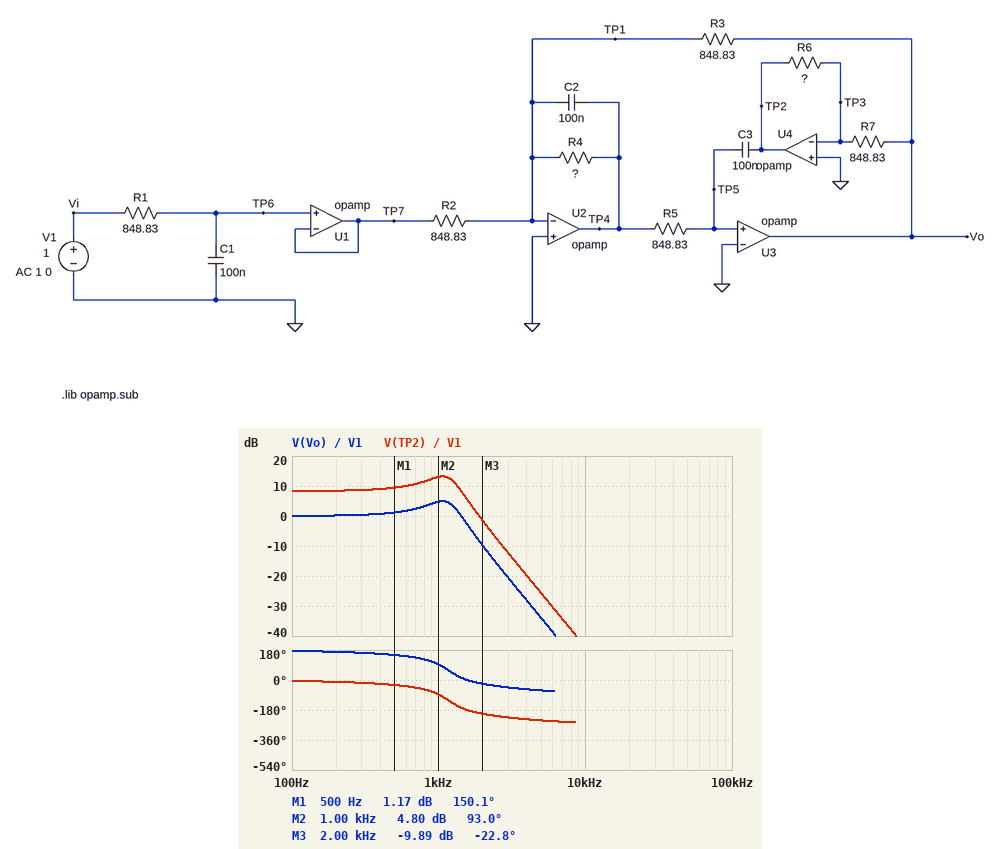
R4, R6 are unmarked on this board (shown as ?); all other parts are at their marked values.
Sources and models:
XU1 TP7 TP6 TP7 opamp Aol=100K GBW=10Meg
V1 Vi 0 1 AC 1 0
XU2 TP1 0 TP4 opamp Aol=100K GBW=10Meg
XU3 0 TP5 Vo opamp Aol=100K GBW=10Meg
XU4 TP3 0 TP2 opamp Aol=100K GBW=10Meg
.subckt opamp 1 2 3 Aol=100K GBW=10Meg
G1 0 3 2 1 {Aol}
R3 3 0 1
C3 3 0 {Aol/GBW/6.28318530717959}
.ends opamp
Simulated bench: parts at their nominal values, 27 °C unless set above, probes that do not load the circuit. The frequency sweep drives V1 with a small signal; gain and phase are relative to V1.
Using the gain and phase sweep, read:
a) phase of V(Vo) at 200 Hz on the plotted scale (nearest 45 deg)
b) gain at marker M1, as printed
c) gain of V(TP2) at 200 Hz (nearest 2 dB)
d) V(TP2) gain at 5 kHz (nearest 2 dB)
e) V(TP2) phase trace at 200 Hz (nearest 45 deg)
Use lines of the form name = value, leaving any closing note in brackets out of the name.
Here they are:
phase of V(Vo) at 200 Hz on the plotted scale = 180 deg
gain at marker M1, as printed = 1.17 dB
gain of V(TP2) at 200 Hz = 8 dB
V(TP2) gain at 5 kHz = -26 dB
V(TP2) phase trace at 200 Hz = 0 deg
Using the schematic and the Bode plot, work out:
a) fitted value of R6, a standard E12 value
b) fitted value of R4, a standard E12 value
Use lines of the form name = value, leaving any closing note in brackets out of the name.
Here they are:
fitted value of R6, a standard E12 value = 2.2 kΩ
fitted value of R4, a standard E12 value = 2.7 kΩ
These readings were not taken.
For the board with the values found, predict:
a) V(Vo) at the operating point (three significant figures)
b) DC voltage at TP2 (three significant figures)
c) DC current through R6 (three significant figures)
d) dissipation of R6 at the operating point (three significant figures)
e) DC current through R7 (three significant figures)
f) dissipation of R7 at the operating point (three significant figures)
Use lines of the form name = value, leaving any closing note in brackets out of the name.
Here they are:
V(Vo) at the operating point = -1.00 V
DC voltage at TP2 = 2.59 V
DC current through R6 = 1.18 mA
dissipation of R6 at the operating point = 3.05 mW
DC current through R7 = 1.18 mA
dissipation of R7 at the operating point = 1.18 mW
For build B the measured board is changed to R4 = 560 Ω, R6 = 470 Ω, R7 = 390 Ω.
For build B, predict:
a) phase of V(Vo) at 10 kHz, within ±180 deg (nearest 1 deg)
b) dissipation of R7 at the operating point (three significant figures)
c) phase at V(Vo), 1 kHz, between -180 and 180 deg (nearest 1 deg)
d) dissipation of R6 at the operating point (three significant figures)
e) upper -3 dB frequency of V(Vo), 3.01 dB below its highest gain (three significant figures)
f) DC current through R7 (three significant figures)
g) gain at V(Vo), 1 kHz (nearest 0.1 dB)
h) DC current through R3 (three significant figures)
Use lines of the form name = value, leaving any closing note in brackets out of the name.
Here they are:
phase of V(Vo) at 10 kHz, within ±180 deg = -63 deg
dissipation of R7 at the operating point = 2.56 mW
phase at V(Vo), 1 kHz, between -180 and 180 deg = 96 deg
dissipation of R6 at the operating point = 3.09 mW
upper -3 dB frequency of V(Vo), 3.01 dB below its highest gain = 1.10 kHz
DC current through R7 = 2.56 mA
gain at V(Vo), 1 kHz = -2.5 dB
DC current through R3 = 1.18 mA
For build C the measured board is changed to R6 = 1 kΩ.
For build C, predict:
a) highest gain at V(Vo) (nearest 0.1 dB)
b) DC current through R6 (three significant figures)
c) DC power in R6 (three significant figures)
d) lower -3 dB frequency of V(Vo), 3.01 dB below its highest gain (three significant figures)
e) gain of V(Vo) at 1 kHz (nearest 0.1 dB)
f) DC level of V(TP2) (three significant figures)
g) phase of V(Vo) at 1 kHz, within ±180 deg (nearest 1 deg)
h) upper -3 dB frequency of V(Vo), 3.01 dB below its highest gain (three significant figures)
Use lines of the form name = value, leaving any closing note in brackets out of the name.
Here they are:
highest gain at V(Vo) = 6.9 dB
DC current through R6 = 1.18 mA
DC power in R6 = 1.39 mW
lower -3 dB frequency of V(Vo), 3.01 dB below its highest gain = 1.26 kHz
gain of V(Vo) at 1 kHz = 2.1 dB
DC level of V(TP2) = 1.18 V
phase of V(Vo) at 1 kHz, within ±180 deg = 135 deg
upper -3 dB frequency of V(Vo), 3.01 dB below its highest gain = 1.92 kHz
